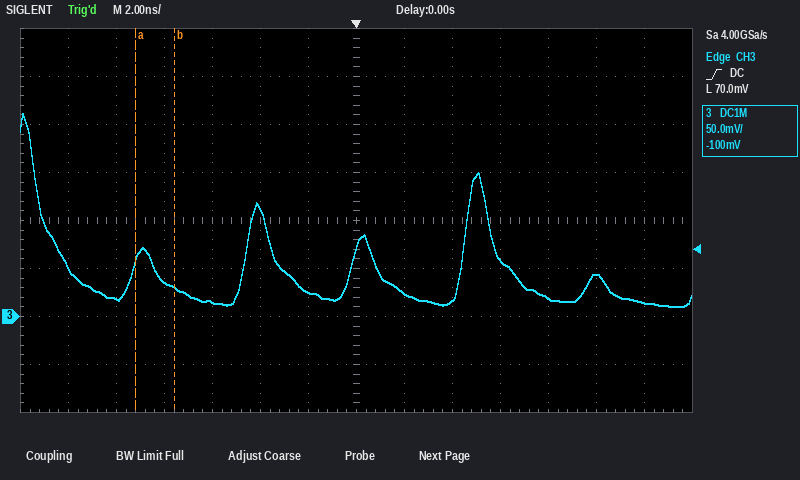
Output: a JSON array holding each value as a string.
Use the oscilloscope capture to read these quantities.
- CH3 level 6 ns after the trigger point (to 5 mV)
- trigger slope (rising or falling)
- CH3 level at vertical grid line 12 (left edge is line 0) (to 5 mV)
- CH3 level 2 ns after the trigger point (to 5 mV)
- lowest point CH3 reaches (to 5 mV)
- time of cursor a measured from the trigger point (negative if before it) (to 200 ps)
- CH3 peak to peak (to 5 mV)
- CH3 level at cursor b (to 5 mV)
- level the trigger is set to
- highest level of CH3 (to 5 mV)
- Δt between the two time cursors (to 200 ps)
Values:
["60 mV", "rising", "45 mV", "25 mV", "10 mV", "-9.2 ns", "200 mV", "30 mV", "70.0 mV", "210 mV", "1.6 ns"]
